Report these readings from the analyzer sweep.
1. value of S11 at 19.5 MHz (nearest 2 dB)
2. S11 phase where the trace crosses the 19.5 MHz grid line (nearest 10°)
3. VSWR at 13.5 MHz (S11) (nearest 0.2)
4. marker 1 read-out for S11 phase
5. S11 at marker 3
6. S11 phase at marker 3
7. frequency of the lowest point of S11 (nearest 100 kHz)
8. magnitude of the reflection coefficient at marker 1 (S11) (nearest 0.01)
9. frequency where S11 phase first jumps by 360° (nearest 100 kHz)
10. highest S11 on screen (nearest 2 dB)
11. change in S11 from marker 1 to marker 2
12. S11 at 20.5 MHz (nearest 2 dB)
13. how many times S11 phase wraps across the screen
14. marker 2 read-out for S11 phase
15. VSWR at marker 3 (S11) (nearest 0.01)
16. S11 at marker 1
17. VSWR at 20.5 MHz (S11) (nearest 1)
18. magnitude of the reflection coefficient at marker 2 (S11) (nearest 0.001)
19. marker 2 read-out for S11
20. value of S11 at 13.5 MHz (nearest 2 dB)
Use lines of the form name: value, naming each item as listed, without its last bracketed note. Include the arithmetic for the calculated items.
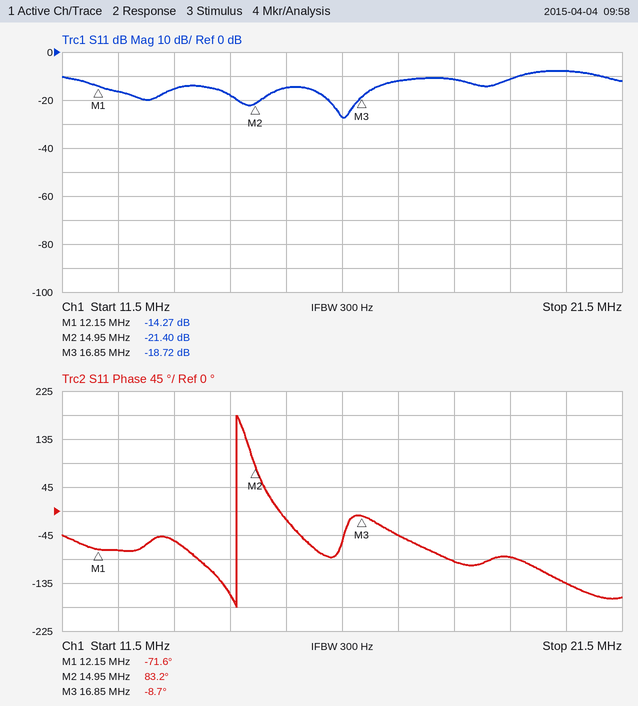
value of S11 at 19.5 MHz: -12 dB
S11 phase where the trace crosses the 19.5 MHz grid line: -90°
VSWR at 13.5 MHz (S11): |Γ| = 10^(-16/20) = 0.1585; VSWR = (1 + 0.1585)/(1 − 0.1585) ≈ 1.4
marker 1 read-out for S11 phase: -71.6°
S11 at marker 3: -18.72 dB
S11 phase at marker 3: -8.7°
frequency of the lowest point of S11: 16.5 MHz
magnitude of the reflection coefficient at marker 1 (S11): 10^(-14.27/20) ≈ 0.19
frequency where S11 phase first jumps by 360°: 14.6 MHz
highest S11 on screen: -8 dB
change in S11 from marker 1 to marker 2: -21.4 − (-14.27) = -7.13 dB
S11 at 20.5 MHz: -8 dB
how many times S11 phase wraps across the screen: 1
marker 2 read-out for S11 phase: 83.2°
VSWR at marker 3 (S11): (1 + 0.1159)/(1 − 0.1159) ≈ 1.26
S11 at marker 1: -14.27 dB
VSWR at 20.5 MHz (S11): |Γ| = 10^(-8/20) = 0.3981; VSWR = (1 + 0.3981)/(1 − 0.3981) ≈ 2
magnitude of the reflection coefficient at marker 2 (S11): 10^(-21.4/20) ≈ 0.085
marker 2 read-out for S11: -21.40 dB
value of S11 at 13.5 MHz: -16 dB
